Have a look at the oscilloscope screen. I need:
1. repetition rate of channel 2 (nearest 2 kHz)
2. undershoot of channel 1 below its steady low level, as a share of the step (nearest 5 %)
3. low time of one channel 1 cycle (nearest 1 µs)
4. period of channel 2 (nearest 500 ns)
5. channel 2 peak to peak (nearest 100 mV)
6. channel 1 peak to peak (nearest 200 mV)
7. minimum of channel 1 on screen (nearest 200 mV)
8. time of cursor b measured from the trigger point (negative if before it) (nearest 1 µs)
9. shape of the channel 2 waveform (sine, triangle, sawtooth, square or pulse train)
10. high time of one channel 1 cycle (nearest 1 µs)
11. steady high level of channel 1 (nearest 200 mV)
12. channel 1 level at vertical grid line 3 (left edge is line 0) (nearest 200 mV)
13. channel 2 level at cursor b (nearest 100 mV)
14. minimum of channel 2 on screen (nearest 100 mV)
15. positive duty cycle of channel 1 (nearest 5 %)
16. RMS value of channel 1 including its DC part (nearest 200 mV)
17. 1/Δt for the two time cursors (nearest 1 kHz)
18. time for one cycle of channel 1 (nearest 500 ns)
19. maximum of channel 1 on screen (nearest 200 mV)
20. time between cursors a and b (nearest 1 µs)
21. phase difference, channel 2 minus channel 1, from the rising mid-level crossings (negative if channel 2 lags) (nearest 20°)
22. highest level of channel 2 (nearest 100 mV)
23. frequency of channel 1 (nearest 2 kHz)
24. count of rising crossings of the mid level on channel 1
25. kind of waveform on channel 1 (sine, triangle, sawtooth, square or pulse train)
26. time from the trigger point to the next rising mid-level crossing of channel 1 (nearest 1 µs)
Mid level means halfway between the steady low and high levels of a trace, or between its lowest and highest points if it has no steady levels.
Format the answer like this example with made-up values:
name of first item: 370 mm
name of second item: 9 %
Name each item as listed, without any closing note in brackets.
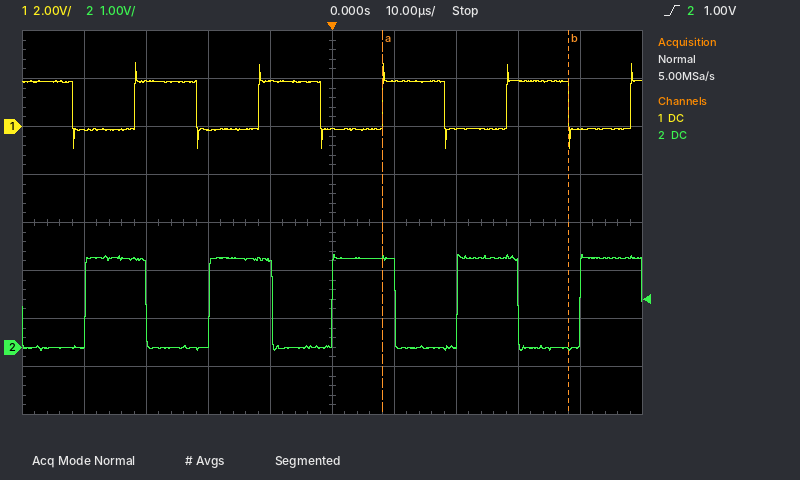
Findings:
repetition rate of channel 2: 50 kHz
undershoot of channel 1 below its steady low level, as a share of the step: 40 %
low time of one channel 1 cycle: 10 µs
period of channel 2: 20.0 µs
channel 2 peak to peak: 2.0 V
channel 1 peak to peak: 3.6 V
minimum of channel 1 on screen: -1.0 V
time of cursor b measured from the trigger point (negative if before it): +38 µs
shape of the channel 2 waveform: square
high time of one channel 1 cycle: 10 µs
steady high level of channel 1: 1.8 V
channel 1 level at vertical grid line 3 (left edge is line 0): -200 mV
channel 2 level at cursor b: 0.0 V
minimum of channel 2 on screen: -100 mV
positive duty cycle of channel 1: 50 %
RMS value of channel 1 including its DC part: 1.4 V
1/Δt for the two time cursors: 33 kHz
time for one cycle of channel 1: 20.0 µs
maximum of channel 1 on screen: 2.6 V
time between cursors a and b: 30 µs
phase difference, channel 2 minus channel 1, from the rising mid-level crossings (negative if channel 2 lags): +140°
highest level of channel 2: 1.9 V
frequency of channel 1: 50 kHz
count of rising crossings of the mid level on channel 1: 5
kind of waveform on channel 1: square
time from the trigger point to the next rising mid-level crossing of channel 1: 8 µs
